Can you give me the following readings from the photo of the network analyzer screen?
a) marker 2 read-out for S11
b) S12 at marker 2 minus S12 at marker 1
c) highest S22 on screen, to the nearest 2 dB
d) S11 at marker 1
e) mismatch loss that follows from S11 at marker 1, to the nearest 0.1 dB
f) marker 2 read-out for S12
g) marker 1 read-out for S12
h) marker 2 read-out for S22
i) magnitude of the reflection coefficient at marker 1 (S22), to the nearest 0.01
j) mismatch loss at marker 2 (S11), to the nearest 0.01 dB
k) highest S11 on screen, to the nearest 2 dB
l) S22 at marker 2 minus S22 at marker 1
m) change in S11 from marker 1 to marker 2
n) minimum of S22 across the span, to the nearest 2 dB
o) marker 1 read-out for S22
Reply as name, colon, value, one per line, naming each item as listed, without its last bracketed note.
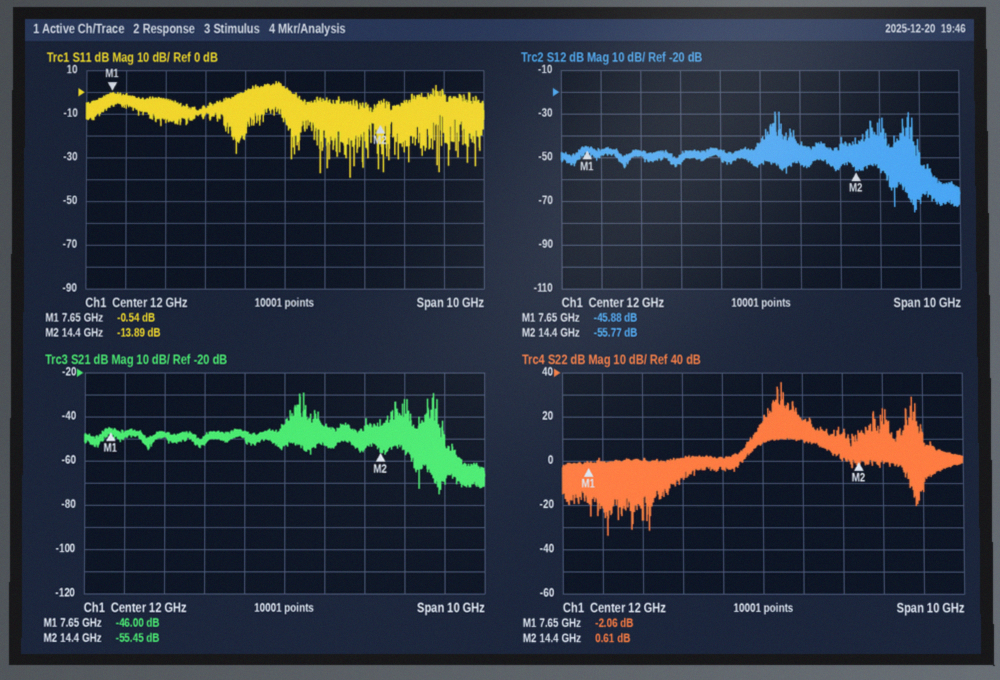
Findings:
marker 2 read-out for S11: -13.89 dB
S12 at marker 2 minus S12 at marker 1: -9.89 dB
highest S22 on screen, to the nearest 2 dB: 36 dB
S11 at marker 1: -0.54 dB
mismatch loss that follows from S11 at marker 1, to the nearest 0.1 dB: 9.3 dB
marker 2 read-out for S12: -55.77 dB
marker 1 read-out for S12: -45.88 dB
marker 2 read-out for S22: 0.61 dB
magnitude of the reflection coefficient at marker 1 (S22), to the nearest 0.01: 0.79
mismatch loss at marker 2 (S11), to the nearest 0.01 dB: 0.18 dB
highest S11 on screen, to the nearest 2 dB: 4 dB
S22 at marker 2 minus S22 at marker 1: 2.67 dB
change in S11 from marker 1 to marker 2: -13.35 dB
minimum of S22 across the span, to the nearest 2 dB: -34 dB
marker 1 read-out for S22: -2.06 dB
